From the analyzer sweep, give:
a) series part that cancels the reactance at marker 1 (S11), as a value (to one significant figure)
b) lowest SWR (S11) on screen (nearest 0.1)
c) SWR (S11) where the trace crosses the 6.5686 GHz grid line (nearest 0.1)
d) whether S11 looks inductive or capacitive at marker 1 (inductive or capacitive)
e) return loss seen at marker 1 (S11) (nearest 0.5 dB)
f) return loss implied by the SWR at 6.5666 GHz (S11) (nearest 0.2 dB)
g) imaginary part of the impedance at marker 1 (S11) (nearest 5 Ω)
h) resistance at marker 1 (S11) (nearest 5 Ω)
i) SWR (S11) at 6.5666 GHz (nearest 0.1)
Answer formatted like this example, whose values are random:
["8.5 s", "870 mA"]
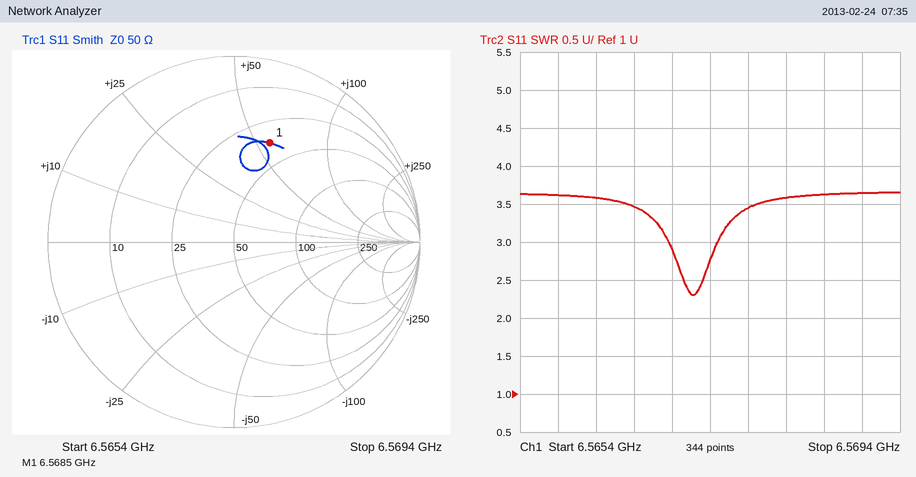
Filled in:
["400 fF", "2.3", "3.6", "inductive", "5.0 dB", "5.2 dB", "+55 Ω", "35 Ω", "3.5"]
